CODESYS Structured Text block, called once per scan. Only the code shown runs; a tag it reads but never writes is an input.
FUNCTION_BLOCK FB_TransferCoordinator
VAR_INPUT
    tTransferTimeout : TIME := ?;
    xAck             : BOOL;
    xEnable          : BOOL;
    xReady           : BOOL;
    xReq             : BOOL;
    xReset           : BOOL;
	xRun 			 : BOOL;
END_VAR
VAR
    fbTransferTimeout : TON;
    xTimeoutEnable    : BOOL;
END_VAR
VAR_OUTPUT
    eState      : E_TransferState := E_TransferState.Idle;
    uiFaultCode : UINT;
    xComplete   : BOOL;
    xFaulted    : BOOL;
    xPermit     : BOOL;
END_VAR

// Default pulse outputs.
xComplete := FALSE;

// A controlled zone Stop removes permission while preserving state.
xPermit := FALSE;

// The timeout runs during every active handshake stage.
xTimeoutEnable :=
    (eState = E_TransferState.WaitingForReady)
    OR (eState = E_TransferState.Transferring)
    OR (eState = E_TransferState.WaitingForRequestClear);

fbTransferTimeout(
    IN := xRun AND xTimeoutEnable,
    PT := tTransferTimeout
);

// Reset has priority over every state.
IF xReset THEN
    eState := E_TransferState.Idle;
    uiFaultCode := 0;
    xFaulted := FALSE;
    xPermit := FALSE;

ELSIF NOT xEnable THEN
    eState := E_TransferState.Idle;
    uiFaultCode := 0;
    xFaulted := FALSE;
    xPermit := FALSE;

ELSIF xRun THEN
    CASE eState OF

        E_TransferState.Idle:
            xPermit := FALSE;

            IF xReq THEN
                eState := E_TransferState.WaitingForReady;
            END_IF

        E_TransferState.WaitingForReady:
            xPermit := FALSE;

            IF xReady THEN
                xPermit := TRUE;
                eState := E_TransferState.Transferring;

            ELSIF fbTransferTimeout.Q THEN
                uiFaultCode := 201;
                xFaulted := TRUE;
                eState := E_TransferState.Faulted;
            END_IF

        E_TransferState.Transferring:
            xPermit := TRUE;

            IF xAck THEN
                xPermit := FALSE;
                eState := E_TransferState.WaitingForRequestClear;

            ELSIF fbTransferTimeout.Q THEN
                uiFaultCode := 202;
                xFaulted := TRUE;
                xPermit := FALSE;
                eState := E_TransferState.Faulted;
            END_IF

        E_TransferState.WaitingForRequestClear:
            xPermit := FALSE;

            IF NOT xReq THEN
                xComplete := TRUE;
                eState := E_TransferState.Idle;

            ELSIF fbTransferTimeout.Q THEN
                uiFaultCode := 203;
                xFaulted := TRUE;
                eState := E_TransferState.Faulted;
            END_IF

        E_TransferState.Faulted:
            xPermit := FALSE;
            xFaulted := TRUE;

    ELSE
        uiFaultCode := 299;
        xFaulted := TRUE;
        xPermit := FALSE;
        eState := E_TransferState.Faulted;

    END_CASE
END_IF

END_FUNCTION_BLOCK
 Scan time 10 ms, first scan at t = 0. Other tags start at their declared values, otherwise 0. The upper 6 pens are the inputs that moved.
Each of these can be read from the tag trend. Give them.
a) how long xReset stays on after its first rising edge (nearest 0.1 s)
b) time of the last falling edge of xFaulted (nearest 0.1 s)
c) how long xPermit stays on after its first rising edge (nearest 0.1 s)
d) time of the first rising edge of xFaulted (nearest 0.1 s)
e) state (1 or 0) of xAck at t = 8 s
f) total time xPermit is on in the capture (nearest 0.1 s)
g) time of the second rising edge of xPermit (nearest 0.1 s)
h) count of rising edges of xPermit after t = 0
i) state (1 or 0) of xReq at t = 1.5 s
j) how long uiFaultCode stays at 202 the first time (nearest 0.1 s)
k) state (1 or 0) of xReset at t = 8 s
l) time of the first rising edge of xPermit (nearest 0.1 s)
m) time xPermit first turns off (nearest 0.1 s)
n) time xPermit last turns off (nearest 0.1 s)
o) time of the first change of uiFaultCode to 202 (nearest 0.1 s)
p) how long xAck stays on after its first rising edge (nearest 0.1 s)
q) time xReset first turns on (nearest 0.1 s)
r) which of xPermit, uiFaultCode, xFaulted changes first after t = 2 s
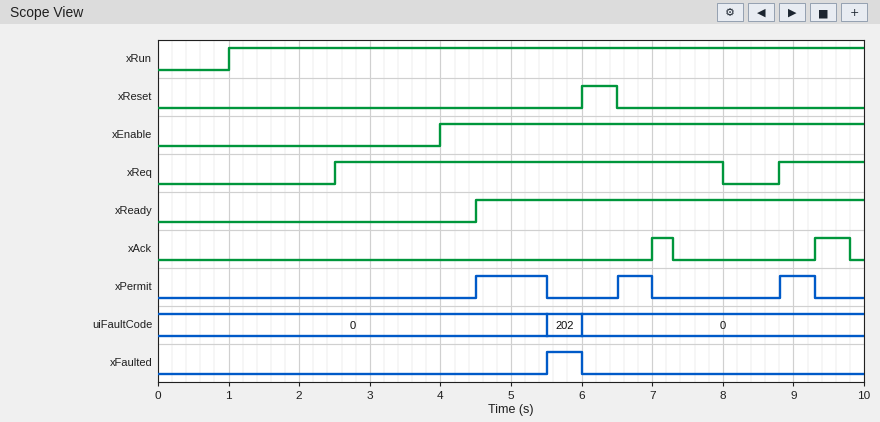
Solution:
0.5 s
6.0 s
1.0 s
5.5 s
0
2.0 s
6.5 s
3
0
0.5 s
0
4.5 s
5.5 s
9.3 s
5.5 s
0.3 s
6.0 s
xPermit
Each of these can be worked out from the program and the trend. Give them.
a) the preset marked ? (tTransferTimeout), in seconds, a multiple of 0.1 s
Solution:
1.5 s
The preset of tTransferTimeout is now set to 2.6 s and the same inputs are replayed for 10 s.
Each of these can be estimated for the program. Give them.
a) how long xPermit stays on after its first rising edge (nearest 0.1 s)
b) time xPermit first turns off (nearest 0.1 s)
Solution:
1.5 s
6.0 s
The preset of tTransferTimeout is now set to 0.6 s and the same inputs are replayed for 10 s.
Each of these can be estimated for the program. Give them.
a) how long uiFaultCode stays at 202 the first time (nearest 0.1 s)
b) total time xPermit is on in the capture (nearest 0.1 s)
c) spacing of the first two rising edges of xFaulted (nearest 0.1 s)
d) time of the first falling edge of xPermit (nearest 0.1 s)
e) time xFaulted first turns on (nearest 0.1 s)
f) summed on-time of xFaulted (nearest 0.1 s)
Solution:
1.4 s
0.6 s
2.5 s
4.6 s
4.6 s
4.3 s
